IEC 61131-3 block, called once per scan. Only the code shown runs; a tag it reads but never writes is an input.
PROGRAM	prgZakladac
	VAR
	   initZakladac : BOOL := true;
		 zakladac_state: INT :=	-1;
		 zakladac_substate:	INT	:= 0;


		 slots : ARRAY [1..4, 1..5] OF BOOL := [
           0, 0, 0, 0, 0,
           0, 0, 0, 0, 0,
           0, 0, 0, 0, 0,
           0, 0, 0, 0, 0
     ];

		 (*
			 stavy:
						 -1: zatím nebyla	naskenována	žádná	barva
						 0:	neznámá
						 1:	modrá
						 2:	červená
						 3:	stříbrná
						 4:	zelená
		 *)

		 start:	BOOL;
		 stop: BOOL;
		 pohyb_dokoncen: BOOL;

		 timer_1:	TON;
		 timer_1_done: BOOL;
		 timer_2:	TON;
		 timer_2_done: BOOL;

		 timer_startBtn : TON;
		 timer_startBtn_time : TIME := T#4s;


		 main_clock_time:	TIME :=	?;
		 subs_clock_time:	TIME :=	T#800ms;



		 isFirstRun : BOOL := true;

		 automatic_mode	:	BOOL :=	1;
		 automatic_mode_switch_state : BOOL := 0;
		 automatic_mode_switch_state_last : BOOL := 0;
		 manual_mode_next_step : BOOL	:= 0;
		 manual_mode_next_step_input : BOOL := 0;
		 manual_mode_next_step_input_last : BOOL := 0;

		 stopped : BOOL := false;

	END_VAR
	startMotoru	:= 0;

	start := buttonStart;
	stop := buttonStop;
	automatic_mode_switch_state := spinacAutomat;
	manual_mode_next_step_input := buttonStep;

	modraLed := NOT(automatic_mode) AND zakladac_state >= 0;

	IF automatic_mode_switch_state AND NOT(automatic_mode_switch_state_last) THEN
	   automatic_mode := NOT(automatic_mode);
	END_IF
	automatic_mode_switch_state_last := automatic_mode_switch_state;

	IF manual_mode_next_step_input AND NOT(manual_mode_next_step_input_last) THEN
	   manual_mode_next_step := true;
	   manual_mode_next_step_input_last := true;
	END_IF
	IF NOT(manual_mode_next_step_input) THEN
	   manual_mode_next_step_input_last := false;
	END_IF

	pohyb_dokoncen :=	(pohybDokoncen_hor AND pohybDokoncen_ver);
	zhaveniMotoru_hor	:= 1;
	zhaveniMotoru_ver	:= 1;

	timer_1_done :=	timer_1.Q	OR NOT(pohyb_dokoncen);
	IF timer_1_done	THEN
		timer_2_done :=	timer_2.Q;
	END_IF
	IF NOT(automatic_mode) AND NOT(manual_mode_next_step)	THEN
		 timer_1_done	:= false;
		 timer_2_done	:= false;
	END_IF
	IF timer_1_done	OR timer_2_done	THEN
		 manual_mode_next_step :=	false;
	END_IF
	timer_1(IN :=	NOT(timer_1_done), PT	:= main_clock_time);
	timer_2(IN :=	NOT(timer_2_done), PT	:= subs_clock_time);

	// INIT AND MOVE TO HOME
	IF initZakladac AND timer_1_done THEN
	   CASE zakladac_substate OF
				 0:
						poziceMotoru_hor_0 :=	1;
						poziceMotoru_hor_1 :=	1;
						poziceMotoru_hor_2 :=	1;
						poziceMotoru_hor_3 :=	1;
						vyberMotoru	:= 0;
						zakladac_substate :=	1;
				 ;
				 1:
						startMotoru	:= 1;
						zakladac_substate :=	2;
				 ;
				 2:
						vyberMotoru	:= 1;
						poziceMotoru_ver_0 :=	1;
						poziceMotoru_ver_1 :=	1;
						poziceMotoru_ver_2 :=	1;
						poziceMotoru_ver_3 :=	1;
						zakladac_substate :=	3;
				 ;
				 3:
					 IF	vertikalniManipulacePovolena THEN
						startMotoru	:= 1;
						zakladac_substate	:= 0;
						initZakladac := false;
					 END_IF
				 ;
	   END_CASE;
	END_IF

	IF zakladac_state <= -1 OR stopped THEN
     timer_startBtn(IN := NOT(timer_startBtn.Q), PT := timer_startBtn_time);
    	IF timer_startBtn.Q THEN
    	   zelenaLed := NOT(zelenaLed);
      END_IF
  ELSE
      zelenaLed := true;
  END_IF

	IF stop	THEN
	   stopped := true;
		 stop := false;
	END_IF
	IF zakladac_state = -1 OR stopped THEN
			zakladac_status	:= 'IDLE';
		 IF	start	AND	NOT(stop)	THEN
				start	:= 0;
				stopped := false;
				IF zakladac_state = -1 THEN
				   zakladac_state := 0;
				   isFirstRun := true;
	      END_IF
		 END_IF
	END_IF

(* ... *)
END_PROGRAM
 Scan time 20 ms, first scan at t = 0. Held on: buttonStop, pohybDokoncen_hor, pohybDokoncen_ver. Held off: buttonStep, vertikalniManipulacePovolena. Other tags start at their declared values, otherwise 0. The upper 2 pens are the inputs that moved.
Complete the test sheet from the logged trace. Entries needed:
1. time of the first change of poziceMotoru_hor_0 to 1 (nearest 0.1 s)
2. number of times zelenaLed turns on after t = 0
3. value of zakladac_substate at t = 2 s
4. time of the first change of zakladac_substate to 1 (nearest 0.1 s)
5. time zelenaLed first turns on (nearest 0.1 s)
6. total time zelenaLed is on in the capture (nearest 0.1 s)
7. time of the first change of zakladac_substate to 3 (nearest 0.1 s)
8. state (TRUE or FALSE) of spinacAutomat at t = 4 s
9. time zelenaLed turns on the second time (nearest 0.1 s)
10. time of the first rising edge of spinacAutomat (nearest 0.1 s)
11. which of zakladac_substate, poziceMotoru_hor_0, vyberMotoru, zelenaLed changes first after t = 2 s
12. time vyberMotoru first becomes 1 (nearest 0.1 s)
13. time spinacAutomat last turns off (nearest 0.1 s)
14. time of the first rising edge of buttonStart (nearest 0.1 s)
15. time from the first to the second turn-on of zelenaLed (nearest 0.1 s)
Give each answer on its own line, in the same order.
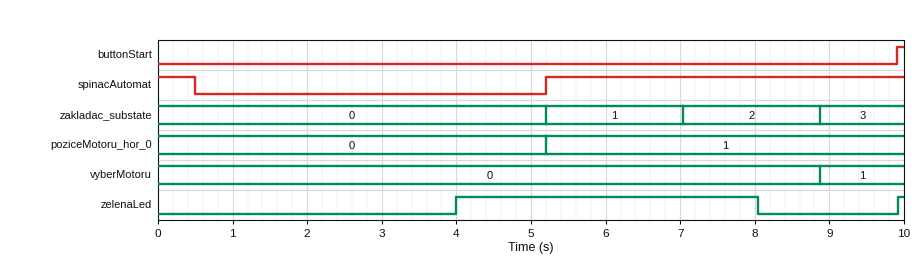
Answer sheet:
5.2 s
2
0
5.2 s
4.0 s
4.1 s
8.9 s
FALSE
9.9 s
5.2 s
zelenaLed
8.9 s
0.5 s
9.9 s
5.9 s
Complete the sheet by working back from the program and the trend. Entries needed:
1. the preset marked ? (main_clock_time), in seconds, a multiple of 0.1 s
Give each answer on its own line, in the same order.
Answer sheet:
1.8 s
